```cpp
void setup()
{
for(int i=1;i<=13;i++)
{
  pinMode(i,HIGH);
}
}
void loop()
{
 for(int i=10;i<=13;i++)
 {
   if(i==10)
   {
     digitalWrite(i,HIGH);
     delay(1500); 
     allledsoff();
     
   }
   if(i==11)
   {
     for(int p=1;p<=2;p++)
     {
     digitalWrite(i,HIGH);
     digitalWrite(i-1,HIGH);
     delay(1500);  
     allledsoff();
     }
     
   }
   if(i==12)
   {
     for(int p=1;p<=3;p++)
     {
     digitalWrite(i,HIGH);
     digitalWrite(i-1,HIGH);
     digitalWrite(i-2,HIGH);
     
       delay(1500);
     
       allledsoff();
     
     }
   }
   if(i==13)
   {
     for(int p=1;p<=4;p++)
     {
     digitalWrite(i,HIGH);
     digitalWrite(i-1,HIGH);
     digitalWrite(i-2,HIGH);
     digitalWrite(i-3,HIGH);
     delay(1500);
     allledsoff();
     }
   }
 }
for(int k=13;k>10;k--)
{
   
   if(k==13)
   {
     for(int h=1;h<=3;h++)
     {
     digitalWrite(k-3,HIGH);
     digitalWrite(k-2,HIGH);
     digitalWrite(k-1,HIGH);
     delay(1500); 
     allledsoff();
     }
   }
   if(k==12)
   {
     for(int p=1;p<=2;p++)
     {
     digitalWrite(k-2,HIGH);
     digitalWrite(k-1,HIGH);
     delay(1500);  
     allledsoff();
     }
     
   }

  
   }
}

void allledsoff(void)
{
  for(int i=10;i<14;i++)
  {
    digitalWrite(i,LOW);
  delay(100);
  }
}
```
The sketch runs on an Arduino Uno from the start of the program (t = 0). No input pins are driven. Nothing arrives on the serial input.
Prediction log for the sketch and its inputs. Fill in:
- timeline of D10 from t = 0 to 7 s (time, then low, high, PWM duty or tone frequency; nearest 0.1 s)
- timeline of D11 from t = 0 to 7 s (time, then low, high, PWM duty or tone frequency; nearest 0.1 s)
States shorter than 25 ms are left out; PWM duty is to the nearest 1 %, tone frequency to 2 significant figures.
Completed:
0 s high; 1.5 s low; 1.9 s high; 3.4 s low; 3.8 s high; 5.3 s low; 5.7 s high
0 s low; 1.9 s high; 3.5 s low; 3.8 s high; 5.4 s low; 5.7 s high
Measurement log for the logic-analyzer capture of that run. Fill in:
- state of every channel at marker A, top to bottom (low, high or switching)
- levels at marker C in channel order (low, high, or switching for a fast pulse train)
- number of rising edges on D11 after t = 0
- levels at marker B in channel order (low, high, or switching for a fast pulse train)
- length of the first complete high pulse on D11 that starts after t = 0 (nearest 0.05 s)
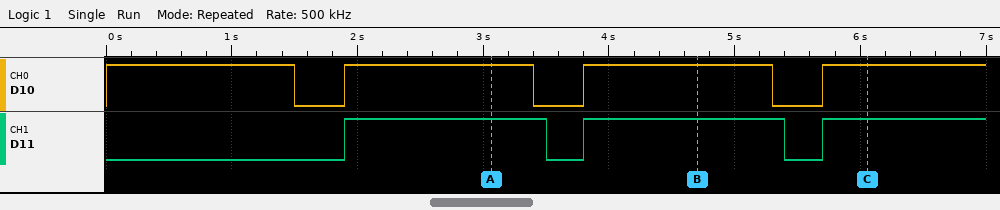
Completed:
D10 high, D11 high
D10 high, D11 high
3
D10 high, D11 high
1.60 s
